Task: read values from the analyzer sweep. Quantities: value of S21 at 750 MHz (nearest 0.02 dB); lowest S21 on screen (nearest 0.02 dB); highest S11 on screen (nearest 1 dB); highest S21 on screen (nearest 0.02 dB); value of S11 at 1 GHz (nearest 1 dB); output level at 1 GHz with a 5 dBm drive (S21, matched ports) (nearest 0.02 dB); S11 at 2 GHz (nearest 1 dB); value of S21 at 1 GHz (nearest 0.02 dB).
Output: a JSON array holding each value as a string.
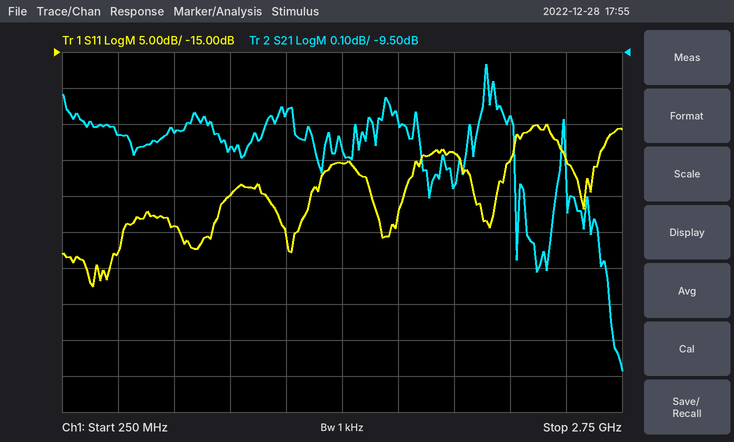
["-9.72 dB", "-10.38 dB", "-25 dB", "-9.54 dB", "-35 dB", "-4.76 dBm", "-29 dB", "-9.76 dB"]
